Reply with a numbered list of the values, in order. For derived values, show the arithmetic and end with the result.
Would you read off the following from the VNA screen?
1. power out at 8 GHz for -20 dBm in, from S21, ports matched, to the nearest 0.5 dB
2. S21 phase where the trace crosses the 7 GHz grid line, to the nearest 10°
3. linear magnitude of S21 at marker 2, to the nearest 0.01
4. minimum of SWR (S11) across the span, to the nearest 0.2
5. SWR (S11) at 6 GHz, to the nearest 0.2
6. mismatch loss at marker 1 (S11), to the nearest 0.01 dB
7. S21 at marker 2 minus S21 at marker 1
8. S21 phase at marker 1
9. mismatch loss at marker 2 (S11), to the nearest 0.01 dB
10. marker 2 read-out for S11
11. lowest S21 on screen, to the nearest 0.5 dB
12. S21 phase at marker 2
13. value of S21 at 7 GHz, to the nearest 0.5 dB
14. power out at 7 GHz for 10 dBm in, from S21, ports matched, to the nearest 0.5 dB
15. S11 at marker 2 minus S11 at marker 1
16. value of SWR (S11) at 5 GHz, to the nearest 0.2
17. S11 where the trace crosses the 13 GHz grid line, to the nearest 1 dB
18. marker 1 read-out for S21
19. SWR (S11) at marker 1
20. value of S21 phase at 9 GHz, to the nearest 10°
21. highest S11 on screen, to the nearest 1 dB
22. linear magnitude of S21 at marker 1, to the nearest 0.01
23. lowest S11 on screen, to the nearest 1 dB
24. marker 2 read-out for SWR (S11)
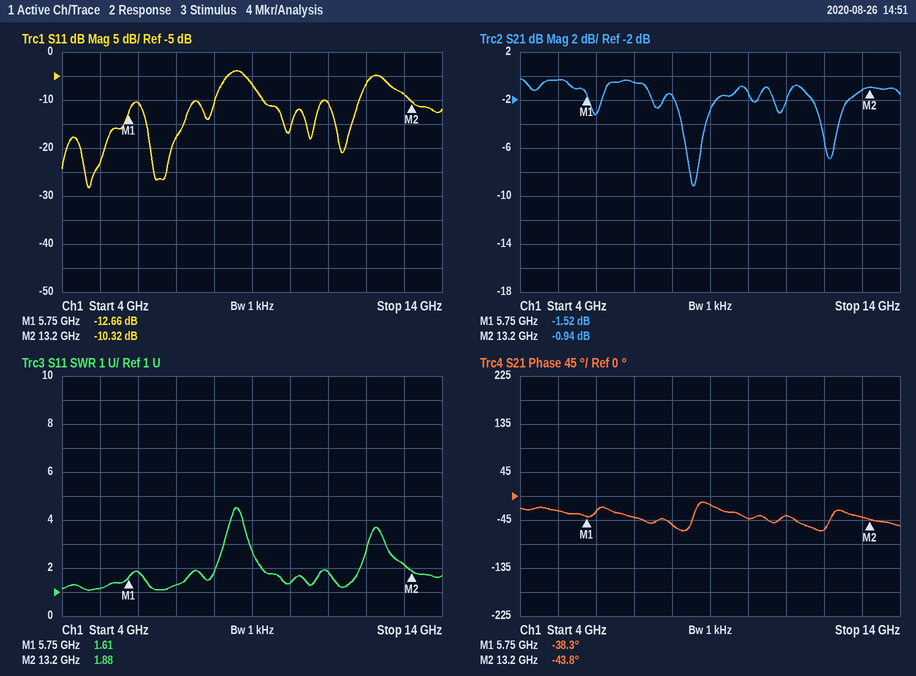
1. -20 dBm + (-1.5 dB) = -21.5 dBm
2. -40°
3. 10^(-0.94/20) ≈ 0.90
4. 1.0
5. 1.8
6. −10 log10(1 − 10^(-12.66/10)) ≈ 0.24 dB
7. -0.94 − (-1.52) = 0.58 dB
8. -38.3°
9. −10 log10(1 − 10^(-10.32/10)) ≈ 0.42 dB
10. -10.32 dB
11. -9.0 dB
12. -43.8°
13. -0.5 dB
14. 10 dBm + (-0.5 dB) = 9.5 dBm
15. -10.32 − (-12.66) = 2.34 dB
16. 1.2
17. -9 dB
18. -1.52 dB
19. 1.61
20. -20°
21. -4 dB
22. 10^(-1.52/20) ≈ 0.84
23. -28 dB
24. 1.88
